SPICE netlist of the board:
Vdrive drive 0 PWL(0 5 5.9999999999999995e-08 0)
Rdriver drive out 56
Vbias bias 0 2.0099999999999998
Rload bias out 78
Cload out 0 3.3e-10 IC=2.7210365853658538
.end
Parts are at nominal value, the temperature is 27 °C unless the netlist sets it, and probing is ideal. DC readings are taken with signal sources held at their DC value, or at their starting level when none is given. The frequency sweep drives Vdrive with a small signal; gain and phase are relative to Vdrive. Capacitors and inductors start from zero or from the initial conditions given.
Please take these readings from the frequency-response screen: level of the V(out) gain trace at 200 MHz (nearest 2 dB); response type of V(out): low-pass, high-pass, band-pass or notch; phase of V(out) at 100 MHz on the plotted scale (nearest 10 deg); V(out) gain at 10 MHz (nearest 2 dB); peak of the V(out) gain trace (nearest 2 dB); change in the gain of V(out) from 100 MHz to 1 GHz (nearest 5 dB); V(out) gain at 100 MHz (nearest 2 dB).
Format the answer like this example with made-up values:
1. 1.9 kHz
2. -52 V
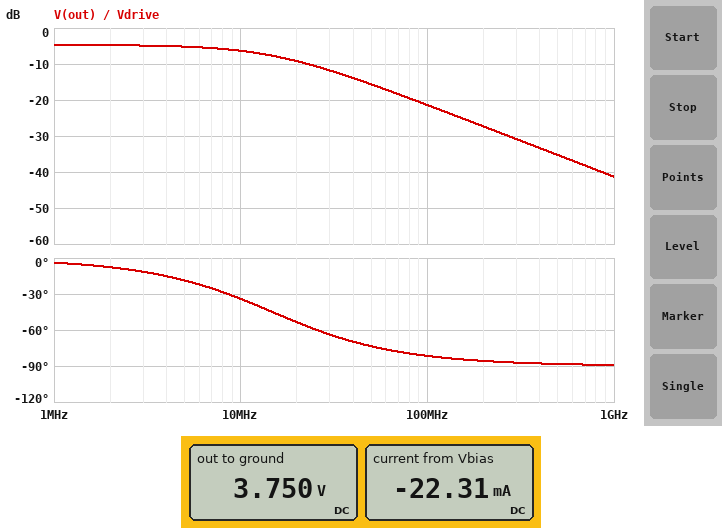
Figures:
1. -28 dB
2. low-pass
3. -80 deg
4. -6 dB
5. -4 dB
6. -20 dB
7. -22 dB
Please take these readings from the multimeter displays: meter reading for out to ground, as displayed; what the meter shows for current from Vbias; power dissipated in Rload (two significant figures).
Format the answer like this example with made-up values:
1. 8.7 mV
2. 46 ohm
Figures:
1. 3.750 V
2. -22.31 mA
3. 39 mW
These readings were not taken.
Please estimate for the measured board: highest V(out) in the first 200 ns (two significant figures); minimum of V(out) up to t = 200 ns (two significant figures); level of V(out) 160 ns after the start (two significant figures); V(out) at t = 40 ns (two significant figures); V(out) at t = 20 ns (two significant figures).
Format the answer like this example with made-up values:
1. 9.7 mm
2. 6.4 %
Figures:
1. 3.2 V
2. 840 mV
3. 840 mV
4. 2.3 V
5. 3.1 V
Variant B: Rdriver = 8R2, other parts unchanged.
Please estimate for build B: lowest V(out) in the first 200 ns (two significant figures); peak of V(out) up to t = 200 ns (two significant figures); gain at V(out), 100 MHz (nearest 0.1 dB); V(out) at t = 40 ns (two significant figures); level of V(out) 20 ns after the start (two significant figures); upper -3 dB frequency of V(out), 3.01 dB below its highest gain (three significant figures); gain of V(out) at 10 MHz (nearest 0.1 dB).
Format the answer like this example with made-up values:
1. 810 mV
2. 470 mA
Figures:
1. 190 mV
2. 4.3 V
3. -6.1 dB
4. 1.9 V
5. 3.4 V
6. 65.0 MHz
7. -1.0 dB
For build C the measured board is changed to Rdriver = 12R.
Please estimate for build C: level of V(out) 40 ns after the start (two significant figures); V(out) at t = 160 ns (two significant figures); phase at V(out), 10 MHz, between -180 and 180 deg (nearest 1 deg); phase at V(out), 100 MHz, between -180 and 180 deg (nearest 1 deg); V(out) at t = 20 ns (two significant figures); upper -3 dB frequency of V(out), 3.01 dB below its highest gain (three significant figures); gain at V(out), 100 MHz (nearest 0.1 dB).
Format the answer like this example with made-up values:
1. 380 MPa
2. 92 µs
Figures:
1. 2.0 V
2. 270 mV
3. -12 deg
4. -65 deg
5. 3.4 V
6. 46.4 MHz
7. -8.8 dB
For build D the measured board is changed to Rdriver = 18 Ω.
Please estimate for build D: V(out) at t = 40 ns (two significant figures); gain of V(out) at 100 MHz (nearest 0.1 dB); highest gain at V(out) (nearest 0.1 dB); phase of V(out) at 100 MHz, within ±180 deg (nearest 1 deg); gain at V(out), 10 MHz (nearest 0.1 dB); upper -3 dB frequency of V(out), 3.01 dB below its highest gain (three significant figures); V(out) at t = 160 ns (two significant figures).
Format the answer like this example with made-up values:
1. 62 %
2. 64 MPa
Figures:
1. 2.1 V
2. -11.9 dB
3. -1.8 dB
4. -72 deg
5. -2.2 dB
6. 33.0 MHz
7. 380 mV
